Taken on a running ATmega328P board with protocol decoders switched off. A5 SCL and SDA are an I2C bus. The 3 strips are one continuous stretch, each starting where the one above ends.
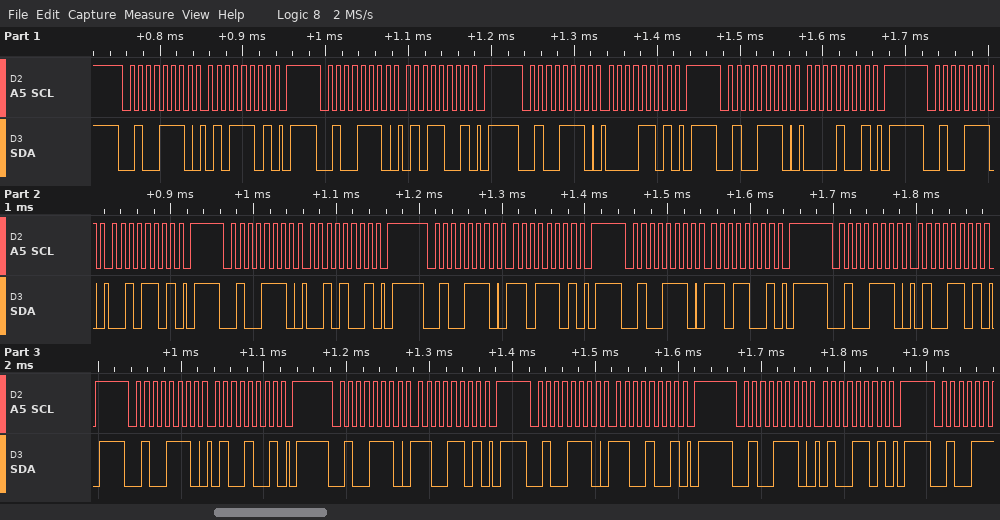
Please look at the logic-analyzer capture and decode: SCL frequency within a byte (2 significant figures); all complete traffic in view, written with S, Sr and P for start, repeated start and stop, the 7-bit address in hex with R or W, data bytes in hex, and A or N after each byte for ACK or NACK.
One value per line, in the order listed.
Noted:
100 kHz
S 27W A 5D A P S 27W A 59 A P S 27W A 0D A P S 27W A 09 A P S 27W A 2D A P S 27W A 29 A P S 27W A DD A P S 27W A D9 A P S 27W A 4D A P S 27W A 49 A P S 27W A CD A P S 27W A C9 A P S 27W A 4D A P
